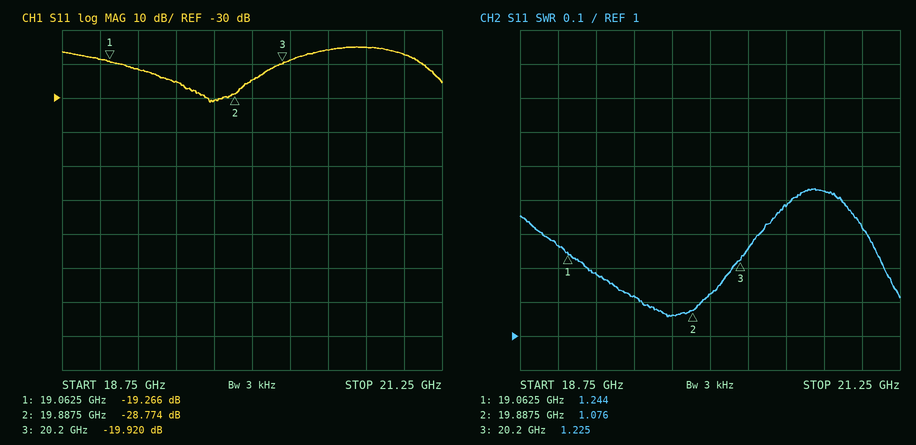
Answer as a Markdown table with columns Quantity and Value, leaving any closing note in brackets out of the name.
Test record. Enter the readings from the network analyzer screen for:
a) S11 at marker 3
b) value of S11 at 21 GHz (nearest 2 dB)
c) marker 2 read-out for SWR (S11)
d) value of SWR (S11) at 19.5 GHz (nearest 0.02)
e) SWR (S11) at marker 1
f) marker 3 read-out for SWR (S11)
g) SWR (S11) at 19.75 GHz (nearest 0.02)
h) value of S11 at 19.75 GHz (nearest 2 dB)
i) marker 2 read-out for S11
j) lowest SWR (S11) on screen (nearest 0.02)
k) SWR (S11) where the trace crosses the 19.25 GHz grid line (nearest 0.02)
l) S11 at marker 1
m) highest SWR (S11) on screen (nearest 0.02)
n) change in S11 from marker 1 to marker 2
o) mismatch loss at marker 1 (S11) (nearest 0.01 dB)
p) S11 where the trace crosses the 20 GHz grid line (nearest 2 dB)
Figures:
| Quantity | Value |
|---|---|
| S11 at marker 3 | -19.920 dB |
| value of S11 at 21 GHz | -18 dB |
| marker 2 read-out for SWR | 1.076 |
| value of SWR (S11) at 19.5 GHz | 1.12 |
| SWR (S11) at marker 1 | 1.244 |
| marker 3 read-out for SWR | 1.225 |
| SWR (S11) at 19.75 GHz | 1.06 |
| value of S11 at 19.75 GHz | -30 dB |
| marker 2 read-out for S11 | -28.774 dB |
| lowest SWR (S11) on screen | 1.06 |
| SWR (S11) where the trace crosses the 19.25 GHz grid line | 1.18 |
| S11 at marker 1 | -19.266 dB |
| highest SWR (S11) on screen | 1.44 |
| change in S11 from marker 1 to marker 2 | -9.508 dB |
| mismatch loss at marker 1 (S11) | 0.05 dB |
| S11 where the trace crosses the 20 GHz grid line | -24 dB |
